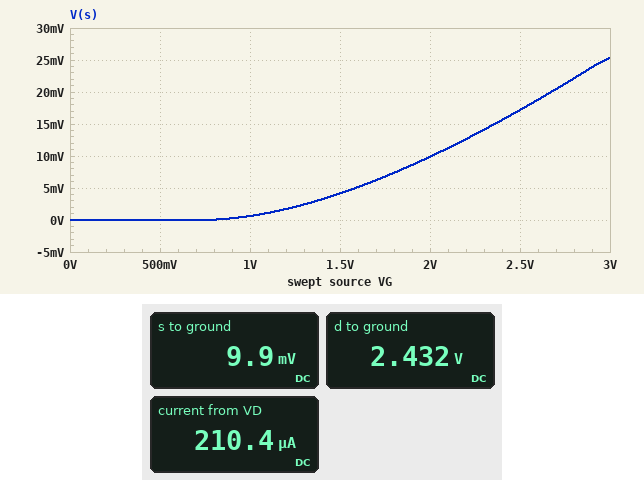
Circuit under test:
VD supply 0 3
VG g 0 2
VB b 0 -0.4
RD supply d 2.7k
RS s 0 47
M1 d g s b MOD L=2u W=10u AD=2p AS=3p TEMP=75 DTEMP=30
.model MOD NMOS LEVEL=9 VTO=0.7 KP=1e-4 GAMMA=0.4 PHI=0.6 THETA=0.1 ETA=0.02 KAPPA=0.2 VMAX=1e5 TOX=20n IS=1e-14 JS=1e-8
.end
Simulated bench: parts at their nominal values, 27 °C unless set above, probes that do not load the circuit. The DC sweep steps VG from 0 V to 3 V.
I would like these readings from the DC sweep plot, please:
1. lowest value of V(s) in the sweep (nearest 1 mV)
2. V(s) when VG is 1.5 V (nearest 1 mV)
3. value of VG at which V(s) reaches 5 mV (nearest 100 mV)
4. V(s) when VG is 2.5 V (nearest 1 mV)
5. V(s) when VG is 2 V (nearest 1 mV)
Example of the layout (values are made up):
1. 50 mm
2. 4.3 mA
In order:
1. 0 V
2. 4 mV
3. 1.6 V
4. 17 mV
5. 10 mV
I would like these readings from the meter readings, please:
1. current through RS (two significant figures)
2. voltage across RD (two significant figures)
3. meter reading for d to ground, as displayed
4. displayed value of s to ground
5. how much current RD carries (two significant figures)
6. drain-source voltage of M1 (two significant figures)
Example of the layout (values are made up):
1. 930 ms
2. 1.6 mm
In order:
1. 210 µA
2. 570 mV
3. 2.432 V
4. 9.9 mV
5. 210 µA
6. 2.4 V
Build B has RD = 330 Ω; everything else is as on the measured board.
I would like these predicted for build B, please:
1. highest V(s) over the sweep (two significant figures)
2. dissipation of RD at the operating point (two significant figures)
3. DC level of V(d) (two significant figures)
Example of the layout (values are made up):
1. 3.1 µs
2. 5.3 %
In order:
1. 26 mV
2. 15 µW
3. 2.9 V
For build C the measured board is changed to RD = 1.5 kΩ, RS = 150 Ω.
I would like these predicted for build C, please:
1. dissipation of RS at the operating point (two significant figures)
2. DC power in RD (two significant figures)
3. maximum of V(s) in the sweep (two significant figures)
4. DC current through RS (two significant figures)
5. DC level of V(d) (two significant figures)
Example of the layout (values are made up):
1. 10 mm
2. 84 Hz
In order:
1. 6.2 µW
2. 62 µW
3. 78 mV
4. 200 µA
5. 2.7 V
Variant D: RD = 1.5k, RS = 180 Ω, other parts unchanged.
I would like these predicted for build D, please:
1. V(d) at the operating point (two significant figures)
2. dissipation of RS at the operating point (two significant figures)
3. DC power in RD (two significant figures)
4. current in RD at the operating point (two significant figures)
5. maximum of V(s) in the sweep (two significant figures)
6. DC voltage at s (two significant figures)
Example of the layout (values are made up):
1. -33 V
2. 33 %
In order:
1. 2.7 V
2. 7.3 µW
3. 61 µW
4. 200 µA
5. 93 mV
6. 36 mV
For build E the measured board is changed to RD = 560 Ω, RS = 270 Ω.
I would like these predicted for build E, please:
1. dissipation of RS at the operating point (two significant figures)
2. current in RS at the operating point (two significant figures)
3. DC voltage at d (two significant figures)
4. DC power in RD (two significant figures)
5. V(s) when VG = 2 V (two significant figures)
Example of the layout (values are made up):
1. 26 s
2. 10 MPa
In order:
1. 10 µW
2. 200 µA
3. 2.9 V
4. 22 µW
5. 53 mV
